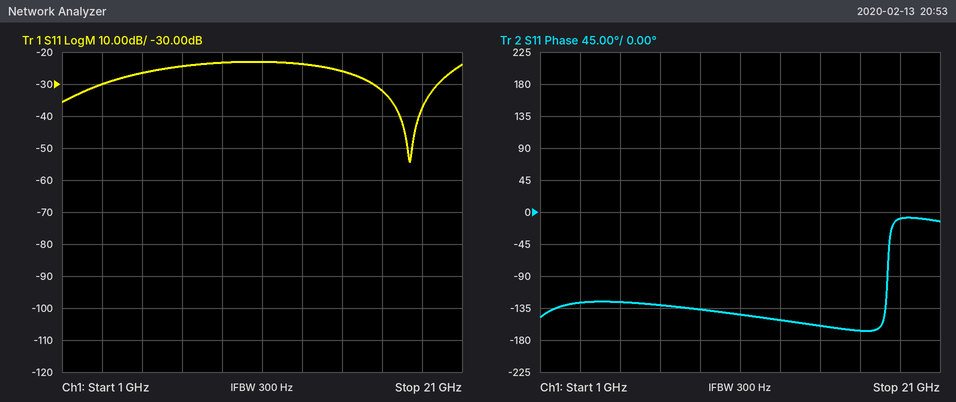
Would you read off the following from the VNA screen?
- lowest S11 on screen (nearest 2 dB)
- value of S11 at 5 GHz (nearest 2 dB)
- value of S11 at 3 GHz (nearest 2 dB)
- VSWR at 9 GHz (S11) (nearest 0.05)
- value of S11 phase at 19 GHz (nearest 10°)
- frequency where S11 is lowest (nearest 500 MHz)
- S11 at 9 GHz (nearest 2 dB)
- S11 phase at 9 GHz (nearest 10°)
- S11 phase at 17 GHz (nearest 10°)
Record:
-54 dB
-26 dB
-30 dB
1.15
-10°
18.5 GHz
-24 dB
-140°
-170°
